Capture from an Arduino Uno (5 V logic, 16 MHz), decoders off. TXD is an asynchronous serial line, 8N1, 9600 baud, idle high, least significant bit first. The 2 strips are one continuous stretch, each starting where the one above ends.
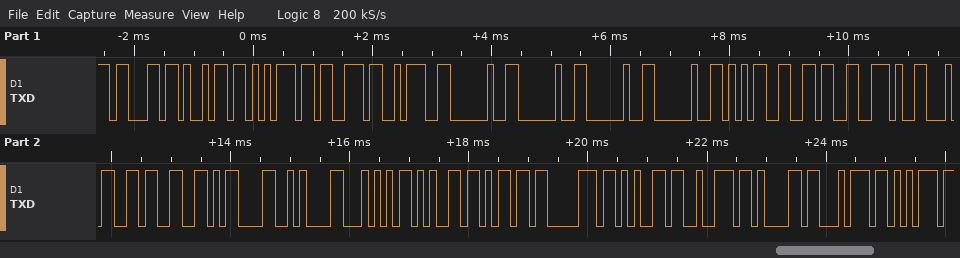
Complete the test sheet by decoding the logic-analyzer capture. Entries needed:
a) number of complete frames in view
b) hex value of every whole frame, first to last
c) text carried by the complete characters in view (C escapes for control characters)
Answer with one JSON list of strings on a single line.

["25", "63 69 75 73 3A 20 20 20 20 35 36 2E 34 33 0D 0A 54 65 6D 70 65 72 61 74 75", "\"cius:    56.43\\r\\nTemperatu\""]
